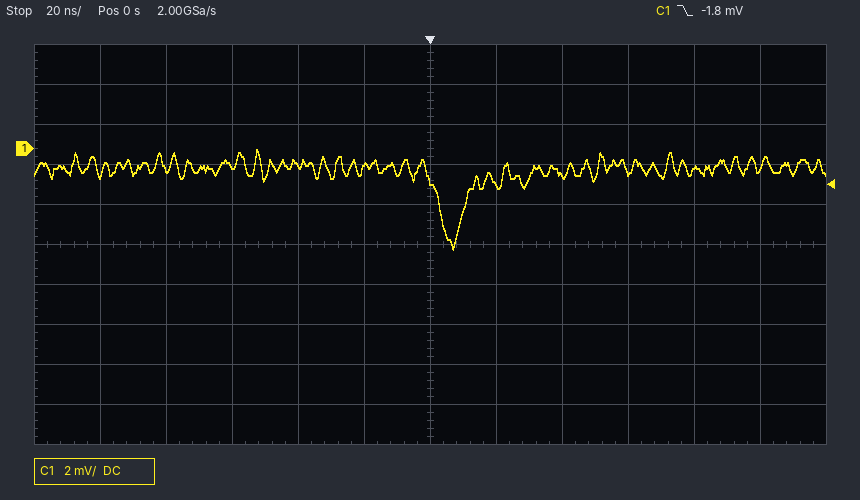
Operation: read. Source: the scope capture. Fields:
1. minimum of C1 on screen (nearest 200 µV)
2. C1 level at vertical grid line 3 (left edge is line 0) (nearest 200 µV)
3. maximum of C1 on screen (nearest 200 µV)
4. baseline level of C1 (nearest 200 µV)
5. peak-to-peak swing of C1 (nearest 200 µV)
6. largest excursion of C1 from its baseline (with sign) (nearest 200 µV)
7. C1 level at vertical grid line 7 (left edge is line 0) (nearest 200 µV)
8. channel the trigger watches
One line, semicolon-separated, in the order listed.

-5.0 mV; -800 µV; 0.0 mV; -1.0 mV; 5.0 mV; -4.0 mV; -1.8 mV; C1
